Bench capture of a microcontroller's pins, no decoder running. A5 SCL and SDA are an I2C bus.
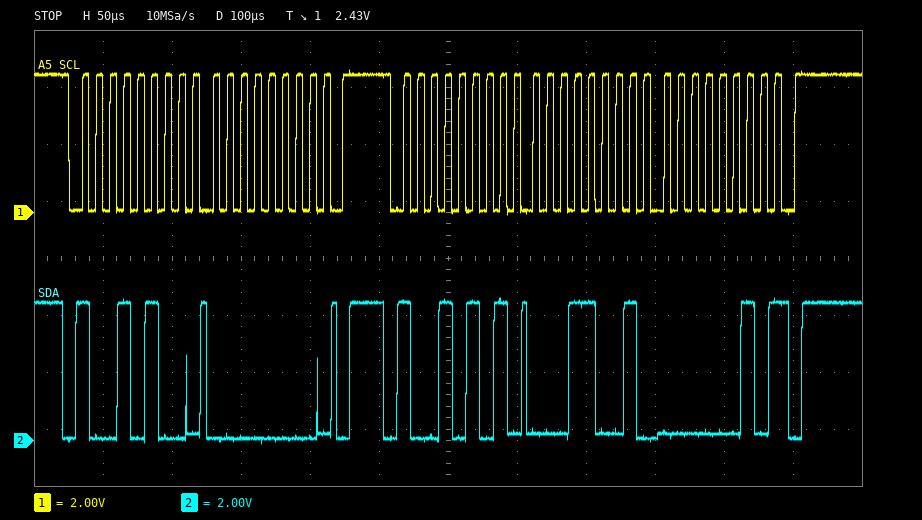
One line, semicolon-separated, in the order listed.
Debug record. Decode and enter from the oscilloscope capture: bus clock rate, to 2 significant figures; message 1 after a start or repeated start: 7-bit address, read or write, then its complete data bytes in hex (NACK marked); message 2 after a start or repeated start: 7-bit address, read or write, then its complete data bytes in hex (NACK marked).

100 kHz; 0x4A write: 00; 0x4A read: 19 02 NACK
